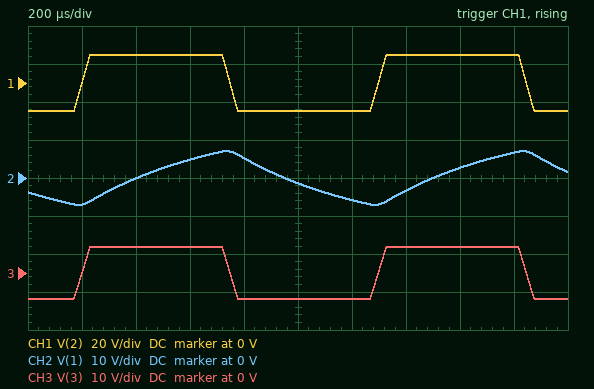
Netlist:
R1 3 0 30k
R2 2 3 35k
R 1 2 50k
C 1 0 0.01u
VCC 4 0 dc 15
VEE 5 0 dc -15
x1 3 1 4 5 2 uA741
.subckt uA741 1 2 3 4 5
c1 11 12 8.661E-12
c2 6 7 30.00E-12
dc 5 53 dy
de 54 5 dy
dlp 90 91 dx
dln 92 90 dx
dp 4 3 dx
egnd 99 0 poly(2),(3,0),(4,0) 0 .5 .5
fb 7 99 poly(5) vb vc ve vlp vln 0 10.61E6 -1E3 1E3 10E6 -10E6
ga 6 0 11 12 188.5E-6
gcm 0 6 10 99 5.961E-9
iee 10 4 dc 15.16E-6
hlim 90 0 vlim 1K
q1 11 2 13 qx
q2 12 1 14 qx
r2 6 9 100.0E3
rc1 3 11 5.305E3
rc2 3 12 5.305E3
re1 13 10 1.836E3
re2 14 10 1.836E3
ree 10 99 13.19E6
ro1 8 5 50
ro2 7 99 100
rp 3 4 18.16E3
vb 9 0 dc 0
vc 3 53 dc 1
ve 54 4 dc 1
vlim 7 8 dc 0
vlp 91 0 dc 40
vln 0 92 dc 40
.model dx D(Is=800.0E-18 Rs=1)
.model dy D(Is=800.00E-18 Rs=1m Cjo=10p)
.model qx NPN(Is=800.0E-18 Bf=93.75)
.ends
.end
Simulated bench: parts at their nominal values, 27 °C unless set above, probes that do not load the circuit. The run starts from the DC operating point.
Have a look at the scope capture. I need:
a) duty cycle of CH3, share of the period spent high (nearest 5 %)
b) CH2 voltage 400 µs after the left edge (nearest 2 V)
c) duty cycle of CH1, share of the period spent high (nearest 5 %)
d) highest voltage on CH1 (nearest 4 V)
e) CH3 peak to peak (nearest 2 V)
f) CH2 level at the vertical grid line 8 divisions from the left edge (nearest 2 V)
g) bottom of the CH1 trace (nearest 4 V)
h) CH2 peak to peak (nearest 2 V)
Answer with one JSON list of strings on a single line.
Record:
["50 %", "0 V", "50 %", "16 V", "14 V", "2 V", "-16 V", "14 V"]
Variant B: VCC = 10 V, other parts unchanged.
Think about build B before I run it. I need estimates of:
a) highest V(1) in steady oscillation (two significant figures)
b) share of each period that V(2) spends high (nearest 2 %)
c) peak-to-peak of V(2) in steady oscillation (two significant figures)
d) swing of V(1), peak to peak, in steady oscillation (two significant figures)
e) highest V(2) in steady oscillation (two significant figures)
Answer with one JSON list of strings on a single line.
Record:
["4.7 V", "56 %", "25 V", "12 V", "9.8 V"]
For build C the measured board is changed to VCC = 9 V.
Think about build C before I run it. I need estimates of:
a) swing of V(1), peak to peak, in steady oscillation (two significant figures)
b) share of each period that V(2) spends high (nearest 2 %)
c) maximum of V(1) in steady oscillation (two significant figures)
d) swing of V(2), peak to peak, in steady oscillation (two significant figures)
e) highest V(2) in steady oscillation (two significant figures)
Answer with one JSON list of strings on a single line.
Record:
["11 V", "58 %", "4.2 V", "24 V", "8.8 V"]
